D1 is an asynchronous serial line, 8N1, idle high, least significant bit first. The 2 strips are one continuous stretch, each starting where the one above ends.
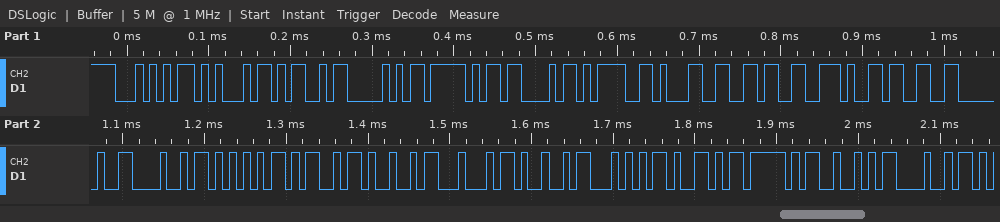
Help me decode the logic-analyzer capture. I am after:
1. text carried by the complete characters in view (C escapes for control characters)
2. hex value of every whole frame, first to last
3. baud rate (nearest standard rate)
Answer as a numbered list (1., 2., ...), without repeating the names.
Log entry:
1. "TEMP_C=16.3 HUMIDITY_RH"
2. 0x54 0x45 0x4D 0x50 0x5F 0x43 0x3D 0x31 0x36 0x2E 0x33 0x20 0x48 0x55 0x4D 0x49 0x44 0x49 0x54 0x59 0x5F 0x52 0x48
3. 115200 baud
